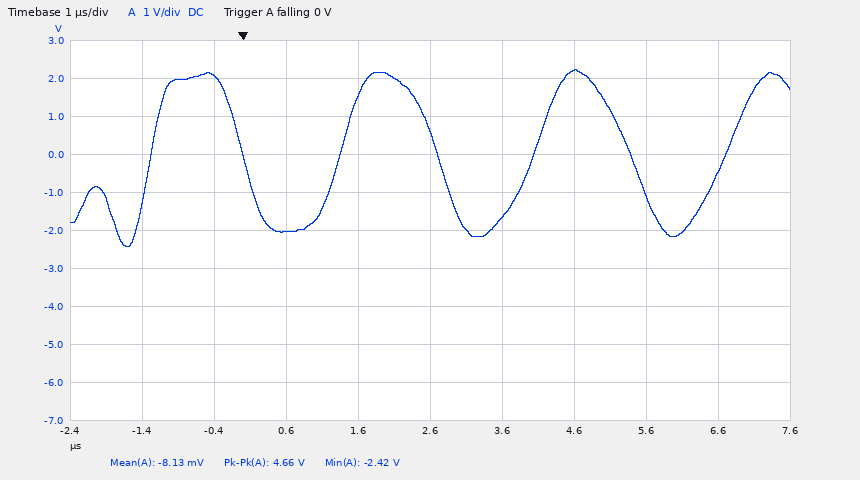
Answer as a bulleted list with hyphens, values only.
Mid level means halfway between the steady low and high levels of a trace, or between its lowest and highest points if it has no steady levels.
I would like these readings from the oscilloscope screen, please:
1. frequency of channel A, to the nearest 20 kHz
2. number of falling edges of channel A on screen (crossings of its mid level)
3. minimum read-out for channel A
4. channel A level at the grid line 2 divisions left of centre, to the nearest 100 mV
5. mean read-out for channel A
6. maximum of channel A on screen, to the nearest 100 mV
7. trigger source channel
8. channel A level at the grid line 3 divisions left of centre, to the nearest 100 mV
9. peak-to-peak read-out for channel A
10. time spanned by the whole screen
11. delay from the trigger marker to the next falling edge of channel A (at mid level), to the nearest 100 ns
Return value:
- 380 kHz
- 3
- -2.42 V
- -2.0 V
- -8.13 mV
- 2.2 V
- channel A
- 2.1 V
- 4.66 V
- 10 µs
- 2.7 µs
